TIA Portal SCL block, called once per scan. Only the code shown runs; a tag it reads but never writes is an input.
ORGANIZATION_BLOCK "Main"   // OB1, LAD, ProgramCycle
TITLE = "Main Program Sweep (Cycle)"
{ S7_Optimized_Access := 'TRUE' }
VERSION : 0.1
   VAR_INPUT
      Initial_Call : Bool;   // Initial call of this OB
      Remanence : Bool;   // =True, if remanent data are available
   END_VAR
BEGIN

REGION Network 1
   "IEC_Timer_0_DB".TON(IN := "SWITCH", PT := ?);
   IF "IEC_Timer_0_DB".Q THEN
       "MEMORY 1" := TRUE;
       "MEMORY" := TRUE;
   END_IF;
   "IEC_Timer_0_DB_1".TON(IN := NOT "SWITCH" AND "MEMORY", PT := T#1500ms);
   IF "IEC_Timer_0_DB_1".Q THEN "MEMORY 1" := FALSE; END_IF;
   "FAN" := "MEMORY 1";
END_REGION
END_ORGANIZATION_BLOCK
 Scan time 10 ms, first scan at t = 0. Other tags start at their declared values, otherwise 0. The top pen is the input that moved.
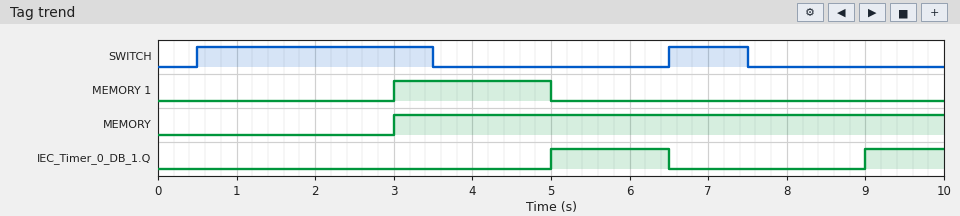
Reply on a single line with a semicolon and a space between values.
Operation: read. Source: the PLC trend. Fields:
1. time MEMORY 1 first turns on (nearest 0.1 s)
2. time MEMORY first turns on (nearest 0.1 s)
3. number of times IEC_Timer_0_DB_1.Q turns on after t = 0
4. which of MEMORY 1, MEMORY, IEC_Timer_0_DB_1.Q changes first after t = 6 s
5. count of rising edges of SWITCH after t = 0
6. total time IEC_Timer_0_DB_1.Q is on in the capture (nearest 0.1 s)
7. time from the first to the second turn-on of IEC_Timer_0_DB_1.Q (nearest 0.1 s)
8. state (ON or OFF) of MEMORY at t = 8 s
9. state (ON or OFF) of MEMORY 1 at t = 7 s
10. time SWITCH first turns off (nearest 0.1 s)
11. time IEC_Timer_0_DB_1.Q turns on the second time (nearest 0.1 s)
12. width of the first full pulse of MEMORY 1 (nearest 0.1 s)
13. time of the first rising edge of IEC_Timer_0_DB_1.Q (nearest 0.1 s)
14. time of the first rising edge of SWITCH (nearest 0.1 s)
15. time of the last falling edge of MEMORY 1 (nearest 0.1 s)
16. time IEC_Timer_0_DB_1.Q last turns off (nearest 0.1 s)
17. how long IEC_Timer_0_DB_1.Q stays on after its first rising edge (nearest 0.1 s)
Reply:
3.0 s; 3.0 s; 2; IEC_Timer_0_DB_1.Q; 2; 2.5 s; 4.0 s; ON; OFF; 3.5 s; 9.0 s; 2.0 s; 5.0 s; 0.5 s; 5.0 s; 6.5 s; 1.5 s
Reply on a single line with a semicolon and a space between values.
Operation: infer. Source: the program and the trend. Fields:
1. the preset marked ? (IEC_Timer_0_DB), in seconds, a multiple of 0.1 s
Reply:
2.5 s
